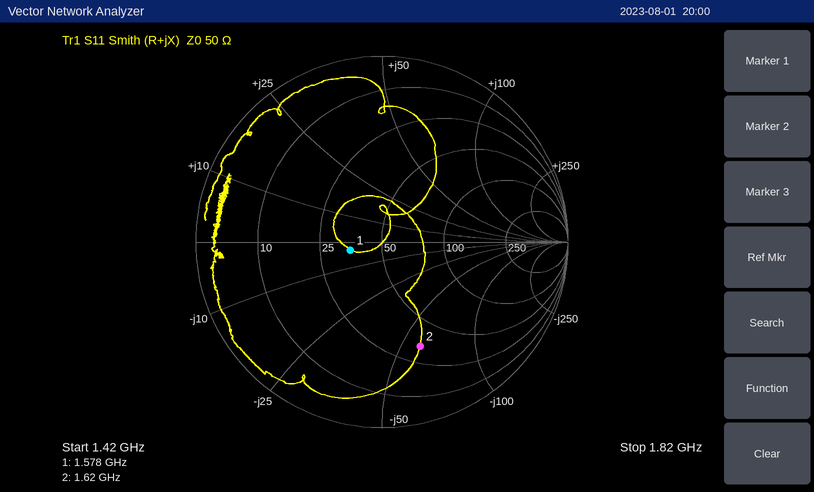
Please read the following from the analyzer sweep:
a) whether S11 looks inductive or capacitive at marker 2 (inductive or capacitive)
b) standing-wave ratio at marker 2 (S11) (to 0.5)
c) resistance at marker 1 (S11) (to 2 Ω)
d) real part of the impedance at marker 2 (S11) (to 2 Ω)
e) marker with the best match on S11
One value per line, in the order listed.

capacitive
4.0
36 Ω
34 Ω
marker 1
